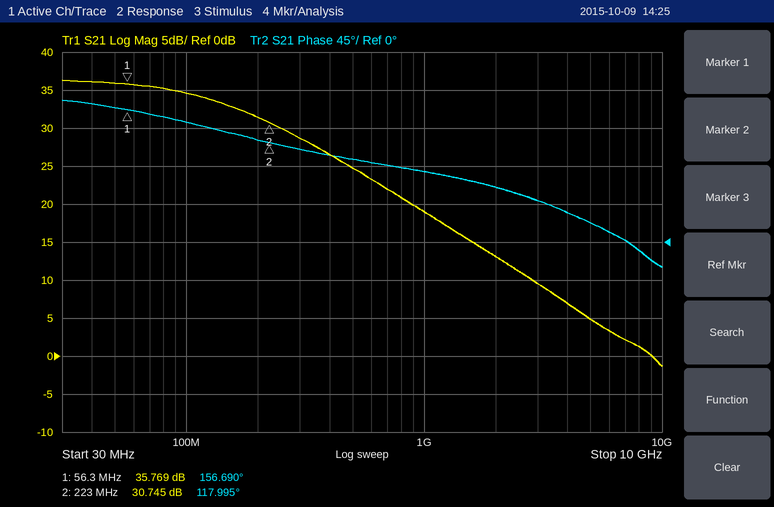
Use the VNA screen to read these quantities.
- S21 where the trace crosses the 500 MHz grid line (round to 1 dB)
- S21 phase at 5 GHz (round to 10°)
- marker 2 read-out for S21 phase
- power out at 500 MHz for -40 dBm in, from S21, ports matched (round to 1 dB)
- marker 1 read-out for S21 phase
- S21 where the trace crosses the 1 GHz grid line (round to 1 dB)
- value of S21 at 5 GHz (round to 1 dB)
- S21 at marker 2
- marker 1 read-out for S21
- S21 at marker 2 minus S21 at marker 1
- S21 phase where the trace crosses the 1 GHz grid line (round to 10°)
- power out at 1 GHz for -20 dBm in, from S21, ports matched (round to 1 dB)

25 dB
20°
117.995°
-15 dBm
156.690°
19 dB
5 dB
30.745 dB
35.769 dB
-5.024 dB
80°
-1 dBm
